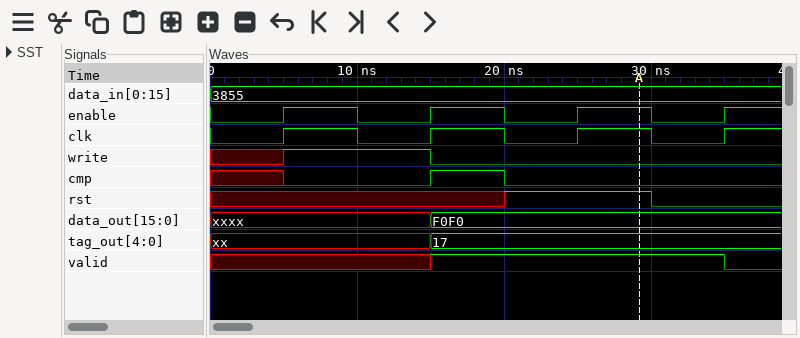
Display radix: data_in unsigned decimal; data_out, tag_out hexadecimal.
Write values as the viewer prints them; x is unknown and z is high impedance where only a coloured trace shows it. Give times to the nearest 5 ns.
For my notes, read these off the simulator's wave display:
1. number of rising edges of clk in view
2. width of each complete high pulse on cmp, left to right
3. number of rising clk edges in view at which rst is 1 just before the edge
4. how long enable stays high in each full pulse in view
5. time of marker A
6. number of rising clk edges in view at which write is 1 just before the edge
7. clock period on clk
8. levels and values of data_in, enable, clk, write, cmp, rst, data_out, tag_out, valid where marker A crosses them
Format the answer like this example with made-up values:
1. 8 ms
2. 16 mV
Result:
1. 4
2. 5 ns
3. 1
4. 5 ns, 5 ns, 5 ns
5. 30 ns
6. 1
7. 10 ns
8. data_in=3855, enable=1, clk=1, write=0, cmp=0, rst=1, data_out=F0F0, tag_out=17, valid=1
